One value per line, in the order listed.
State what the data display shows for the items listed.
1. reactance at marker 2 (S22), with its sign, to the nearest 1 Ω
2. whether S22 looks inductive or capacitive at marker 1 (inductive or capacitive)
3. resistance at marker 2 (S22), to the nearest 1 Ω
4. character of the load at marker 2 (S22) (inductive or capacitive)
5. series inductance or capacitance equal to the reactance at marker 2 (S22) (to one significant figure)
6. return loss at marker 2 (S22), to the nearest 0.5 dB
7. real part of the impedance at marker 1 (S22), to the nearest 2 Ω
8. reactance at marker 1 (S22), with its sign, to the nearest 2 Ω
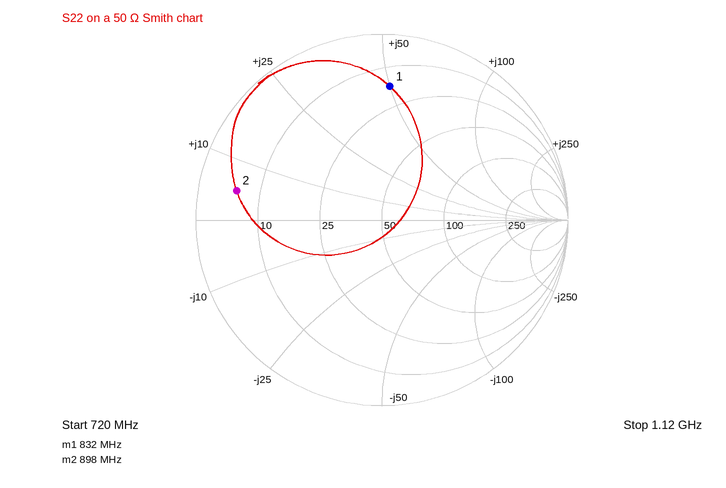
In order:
+5 Ω
inductive
6 Ω
inductive
900 pH
2.0 dB
16 Ω
+50 Ω
